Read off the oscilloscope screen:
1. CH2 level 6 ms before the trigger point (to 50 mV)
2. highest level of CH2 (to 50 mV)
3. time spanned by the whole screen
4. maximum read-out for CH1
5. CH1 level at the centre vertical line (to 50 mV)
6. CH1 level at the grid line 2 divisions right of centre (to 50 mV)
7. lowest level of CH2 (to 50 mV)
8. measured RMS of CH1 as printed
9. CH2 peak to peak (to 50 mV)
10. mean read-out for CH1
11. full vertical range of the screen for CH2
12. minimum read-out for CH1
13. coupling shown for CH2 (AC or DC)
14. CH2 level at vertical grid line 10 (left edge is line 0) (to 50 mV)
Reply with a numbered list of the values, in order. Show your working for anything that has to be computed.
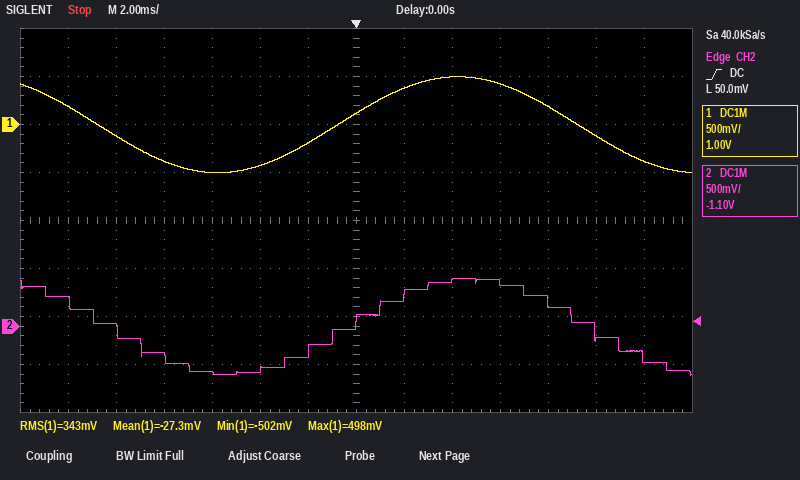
1. -500 mV
2. 500 mV
3. 28 ms
4. 498 mV
5. 100 mV
6. 500 mV
7. -500 mV
8. 343 mV
9. 500 mV − (-500 mV) = 1.00 V
10. -27.3 mV
11. 4 V
12. -502 mV
13. DC
14. 450 mV
